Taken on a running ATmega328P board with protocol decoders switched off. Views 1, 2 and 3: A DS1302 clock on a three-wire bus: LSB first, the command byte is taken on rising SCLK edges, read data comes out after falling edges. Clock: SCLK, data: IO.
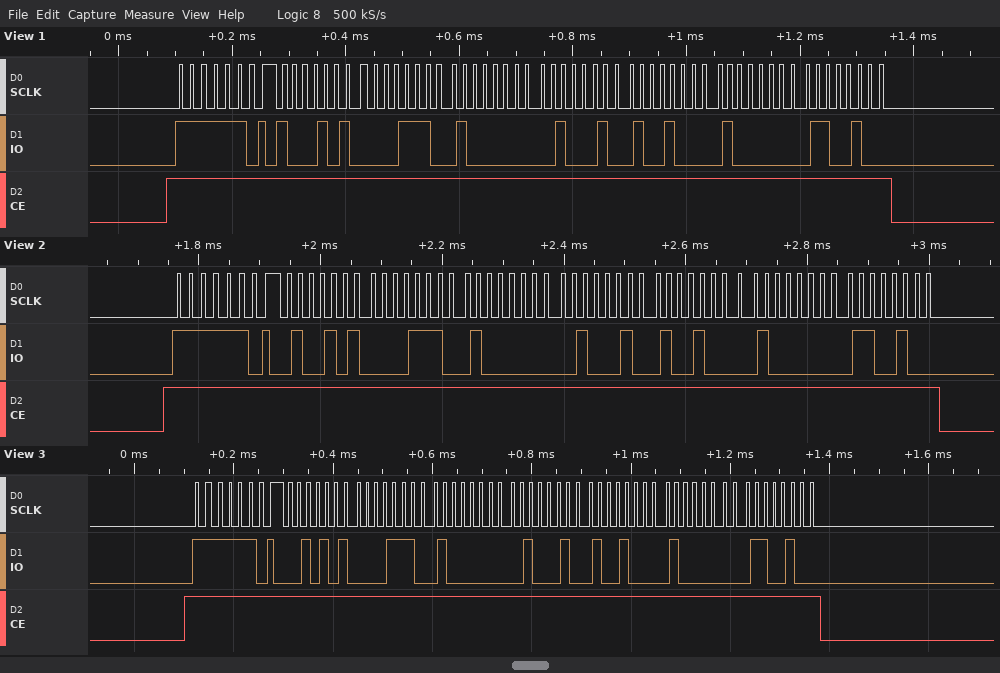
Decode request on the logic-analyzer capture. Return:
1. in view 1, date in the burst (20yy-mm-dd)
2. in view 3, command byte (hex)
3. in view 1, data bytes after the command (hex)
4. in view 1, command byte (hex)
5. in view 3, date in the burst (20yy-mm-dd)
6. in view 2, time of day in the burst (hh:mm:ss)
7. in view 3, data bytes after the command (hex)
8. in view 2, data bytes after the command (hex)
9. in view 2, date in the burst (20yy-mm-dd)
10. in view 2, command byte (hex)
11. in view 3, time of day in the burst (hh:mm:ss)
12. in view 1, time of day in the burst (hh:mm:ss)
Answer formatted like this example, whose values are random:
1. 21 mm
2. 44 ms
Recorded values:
1. 2013-09-22
2. 0xBF
3. 51 38 01 22 09 01 13
4. 0xBF
5. 2013-09-22
6. 01:38:52
7. 54 38 01 22 09 01 13
8. 52 38 01 22 09 01 13
9. 2013-09-22
10. 0xBF
11. 01:38:54
12. 01:38:51
